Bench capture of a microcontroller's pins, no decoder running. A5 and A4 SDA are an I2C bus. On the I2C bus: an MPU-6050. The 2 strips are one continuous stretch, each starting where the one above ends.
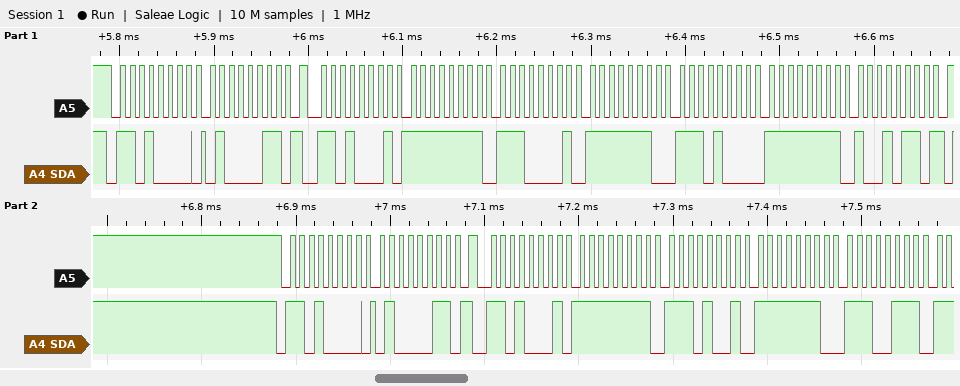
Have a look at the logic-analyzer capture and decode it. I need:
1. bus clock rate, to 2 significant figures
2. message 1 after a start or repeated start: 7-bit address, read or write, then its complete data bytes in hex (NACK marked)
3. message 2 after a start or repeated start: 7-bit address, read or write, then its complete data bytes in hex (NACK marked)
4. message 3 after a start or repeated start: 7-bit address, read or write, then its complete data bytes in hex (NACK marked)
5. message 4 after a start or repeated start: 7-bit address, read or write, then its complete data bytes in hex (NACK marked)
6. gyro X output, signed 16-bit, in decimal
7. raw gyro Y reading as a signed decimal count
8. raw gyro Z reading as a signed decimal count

100 kHz
0x68 write: 43
0x68 read: FF E1 FE E8 FF 96 NACK
0x68 write: 43
0x68 read: FF E9 FE E7
-31
-280
-106
